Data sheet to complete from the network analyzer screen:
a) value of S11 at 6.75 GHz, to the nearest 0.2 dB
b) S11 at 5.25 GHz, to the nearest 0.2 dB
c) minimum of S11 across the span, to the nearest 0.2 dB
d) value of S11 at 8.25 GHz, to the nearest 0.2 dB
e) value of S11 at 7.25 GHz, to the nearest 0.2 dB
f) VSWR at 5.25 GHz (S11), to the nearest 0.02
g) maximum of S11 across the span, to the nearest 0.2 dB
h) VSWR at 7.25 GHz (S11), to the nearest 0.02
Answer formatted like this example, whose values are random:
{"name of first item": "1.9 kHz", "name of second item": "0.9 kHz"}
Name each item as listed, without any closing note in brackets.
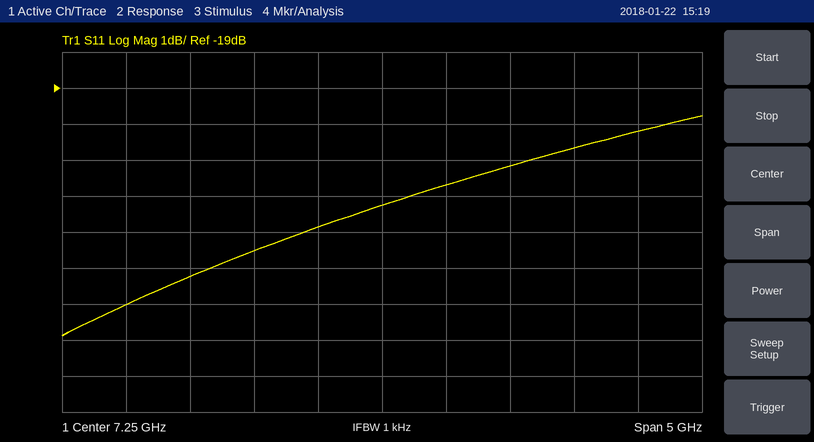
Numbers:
{"value of S11 at 6.75 GHz, to the nearest 0.2 dB": "-22.8 dB", "S11 at 5.25 GHz, to the nearest 0.2 dB": "-25.0 dB", "minimum of S11 across the span, to the nearest 0.2 dB": "-25.8 dB", "value of S11 at 8.25 GHz, to the nearest 0.2 dB": "-21.2 dB", "value of S11 at 7.25 GHz, to the nearest 0.2 dB": "-22.2 dB", "VSWR at 5.25 GHz (S11), to the nearest 0.02": "1.12", "maximum of S11 across the span, to the nearest 0.2 dB": "-19.8 dB", "VSWR at 7.25 GHz (S11), to the nearest 0.02": "1.16"}
